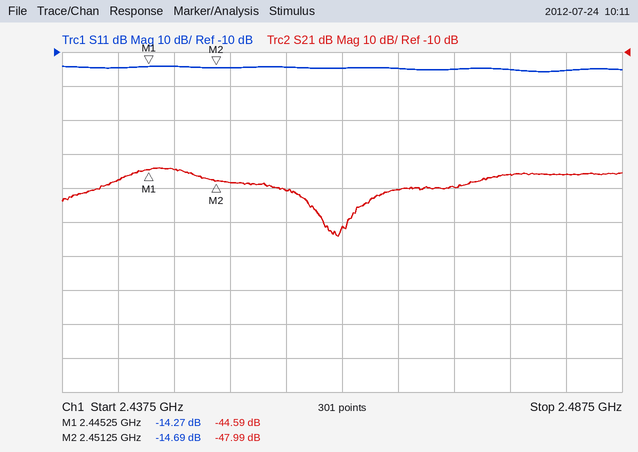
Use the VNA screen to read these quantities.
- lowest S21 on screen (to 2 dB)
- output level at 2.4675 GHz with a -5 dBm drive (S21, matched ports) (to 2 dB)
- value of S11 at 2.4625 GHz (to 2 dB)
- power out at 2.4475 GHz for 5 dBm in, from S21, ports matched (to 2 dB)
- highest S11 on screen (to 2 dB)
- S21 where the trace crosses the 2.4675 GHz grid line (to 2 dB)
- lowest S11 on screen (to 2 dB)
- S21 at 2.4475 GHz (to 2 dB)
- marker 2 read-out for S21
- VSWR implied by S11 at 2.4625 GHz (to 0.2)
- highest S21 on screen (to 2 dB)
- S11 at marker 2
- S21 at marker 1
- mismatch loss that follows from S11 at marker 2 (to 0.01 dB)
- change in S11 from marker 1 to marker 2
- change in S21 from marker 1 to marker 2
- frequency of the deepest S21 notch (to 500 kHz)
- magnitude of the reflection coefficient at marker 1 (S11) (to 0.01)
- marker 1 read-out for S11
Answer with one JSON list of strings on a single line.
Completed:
["-64 dB", "-56 dBm", "-14 dB", "-40 dBm", "-14 dB", "-50 dB", "-16 dB", "-44 dB", "-47.99 dB", "1.4", "-44 dB", "-14.69 dB", "-44.59 dB", "0.15 dB", "-0.42 dB", "-3.40 dB", "2.4620 GHz", "0.19", "-14.27 dB"]
